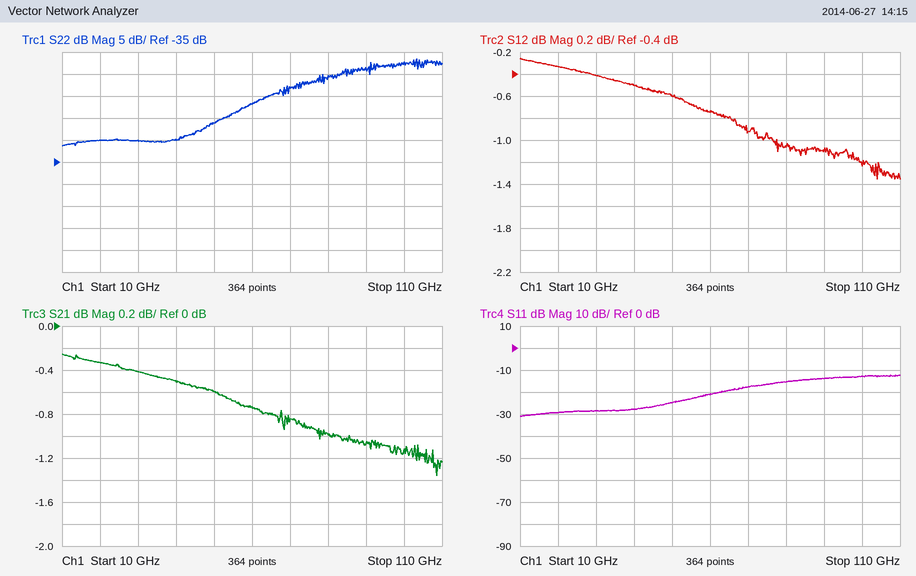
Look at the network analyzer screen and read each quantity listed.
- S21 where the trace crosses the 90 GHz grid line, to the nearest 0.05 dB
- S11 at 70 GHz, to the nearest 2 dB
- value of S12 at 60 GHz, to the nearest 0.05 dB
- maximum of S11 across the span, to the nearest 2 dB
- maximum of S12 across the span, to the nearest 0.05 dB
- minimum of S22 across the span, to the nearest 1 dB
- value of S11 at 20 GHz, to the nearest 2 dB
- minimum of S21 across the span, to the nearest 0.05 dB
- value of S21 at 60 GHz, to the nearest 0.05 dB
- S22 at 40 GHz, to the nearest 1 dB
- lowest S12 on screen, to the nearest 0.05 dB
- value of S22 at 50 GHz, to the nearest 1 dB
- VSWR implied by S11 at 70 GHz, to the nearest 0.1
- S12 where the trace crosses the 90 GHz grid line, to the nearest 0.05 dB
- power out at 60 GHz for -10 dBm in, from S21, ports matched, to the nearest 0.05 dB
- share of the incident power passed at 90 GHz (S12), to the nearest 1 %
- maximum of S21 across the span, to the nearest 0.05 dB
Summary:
-1.05 dB
-18 dB
-0.75 dB
-12 dB
-0.25 dB
-31 dB
-30 dB
-1.35 dB
-0.75 dB
-30 dB
-1.35 dB
-26 dB
1.3
-1.10 dB
-10.75 dBm
78 %
-0.25 dB
